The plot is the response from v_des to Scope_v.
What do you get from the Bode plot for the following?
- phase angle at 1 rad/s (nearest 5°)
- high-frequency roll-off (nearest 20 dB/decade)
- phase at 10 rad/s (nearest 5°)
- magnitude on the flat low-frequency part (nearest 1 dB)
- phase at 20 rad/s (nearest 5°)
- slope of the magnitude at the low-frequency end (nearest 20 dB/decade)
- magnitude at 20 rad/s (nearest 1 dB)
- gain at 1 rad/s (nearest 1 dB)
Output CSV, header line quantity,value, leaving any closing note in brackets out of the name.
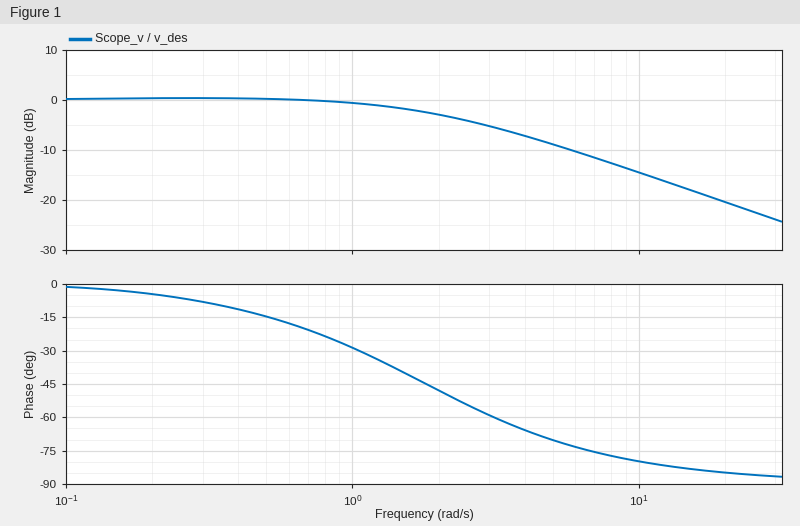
quantity,value
phase angle at 1 rad/s,-30°
high-frequency roll-off,-20 dB/decade
phase at 10 rad/s,-80°
magnitude on the flat low-frequency part,0 dB
phase at 20 rad/s,-85°
slope of the magnitude at the low-frequency end,0 dB/decade
magnitude at 20 rad/s,-20 dB
gain at 1 rad/s,-1 dB
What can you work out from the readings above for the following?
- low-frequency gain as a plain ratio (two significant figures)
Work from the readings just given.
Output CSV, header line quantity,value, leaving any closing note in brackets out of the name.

quantity,value
low-frequency gain as a plain ratio,1.0
